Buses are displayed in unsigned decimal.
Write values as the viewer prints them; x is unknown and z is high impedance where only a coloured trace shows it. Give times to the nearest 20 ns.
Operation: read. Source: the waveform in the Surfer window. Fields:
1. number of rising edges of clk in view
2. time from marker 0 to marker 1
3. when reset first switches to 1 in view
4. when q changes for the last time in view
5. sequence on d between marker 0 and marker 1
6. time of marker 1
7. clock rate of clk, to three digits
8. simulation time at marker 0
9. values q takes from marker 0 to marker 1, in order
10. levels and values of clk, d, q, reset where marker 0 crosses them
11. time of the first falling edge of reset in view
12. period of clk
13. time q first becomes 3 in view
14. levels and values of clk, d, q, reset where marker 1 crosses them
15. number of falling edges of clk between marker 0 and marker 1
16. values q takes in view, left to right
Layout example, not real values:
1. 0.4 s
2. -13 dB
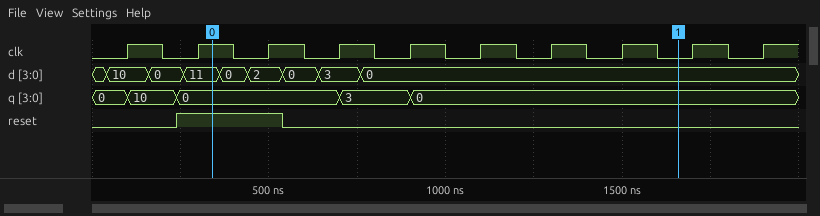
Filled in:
1. 10
2. 1320 ns
3. 240 ns
4. 900 ns
5. 11, 0, 2, 0, 3, 0
6. 1660 ns
7. 5.00 MHz
8. 340 ns
9. 0, 3, 0
10. clk=1, d=11, q=0, reset=1
11. 540 ns
12. 200 ns
13. 700 ns
14. clk=0, d=0, q=0, reset=0
15. 7
16. 0, 10, 0, 3, 0
